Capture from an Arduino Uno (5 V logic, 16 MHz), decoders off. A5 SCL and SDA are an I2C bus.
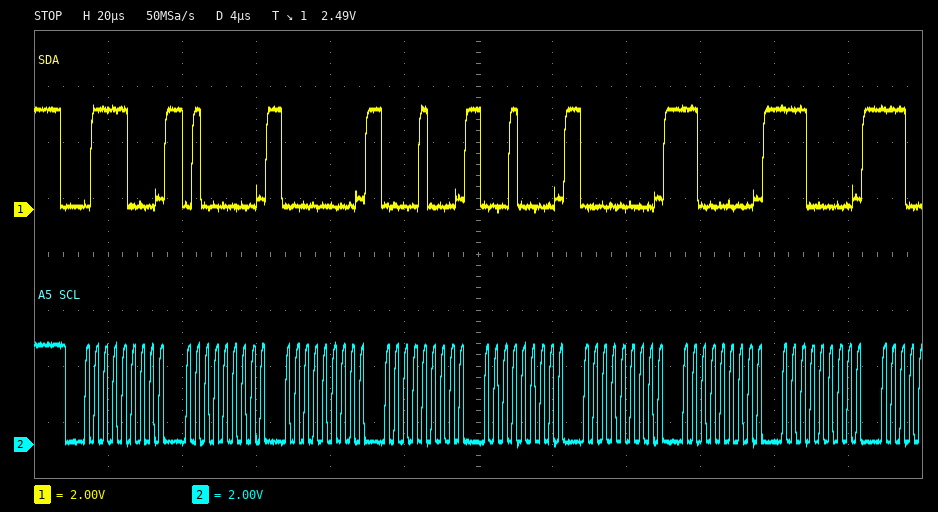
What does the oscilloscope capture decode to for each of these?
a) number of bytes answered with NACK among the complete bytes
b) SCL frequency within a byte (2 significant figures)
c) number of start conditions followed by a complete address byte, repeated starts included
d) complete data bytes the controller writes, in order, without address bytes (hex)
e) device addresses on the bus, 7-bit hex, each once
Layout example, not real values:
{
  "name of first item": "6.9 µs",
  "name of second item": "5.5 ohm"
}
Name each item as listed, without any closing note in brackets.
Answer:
{
  "number of bytes answered with NACK among the complete bytes": "0",
  "SCL frequency within a byte": "400 kHz",
  "number of start conditions followed by a complete address byte, repeated starts included": "1",
  "complete data bytes the controller writes, in order, without address bytes": "40 00 08 10 00 C0 E0",
  "device addresses on the bus, 7-bit hex, each once": "0x3C"
}
